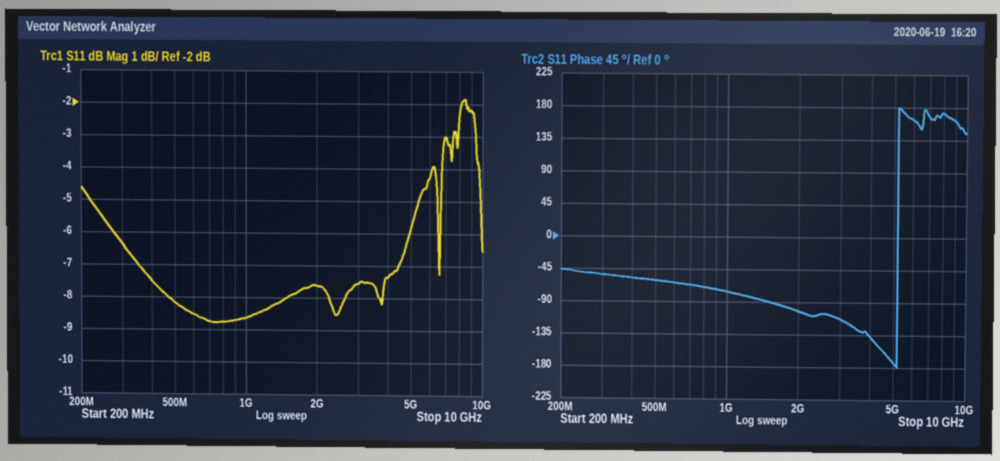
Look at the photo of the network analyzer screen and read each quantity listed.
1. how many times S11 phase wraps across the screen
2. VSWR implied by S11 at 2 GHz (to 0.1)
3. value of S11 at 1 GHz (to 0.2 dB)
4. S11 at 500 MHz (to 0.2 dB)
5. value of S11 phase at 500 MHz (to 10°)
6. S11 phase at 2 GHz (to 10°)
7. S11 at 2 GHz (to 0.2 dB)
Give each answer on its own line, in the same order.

1
2.4
-8.6 dB
-8.2 dB
-60°
-100°
-7.6 dB
